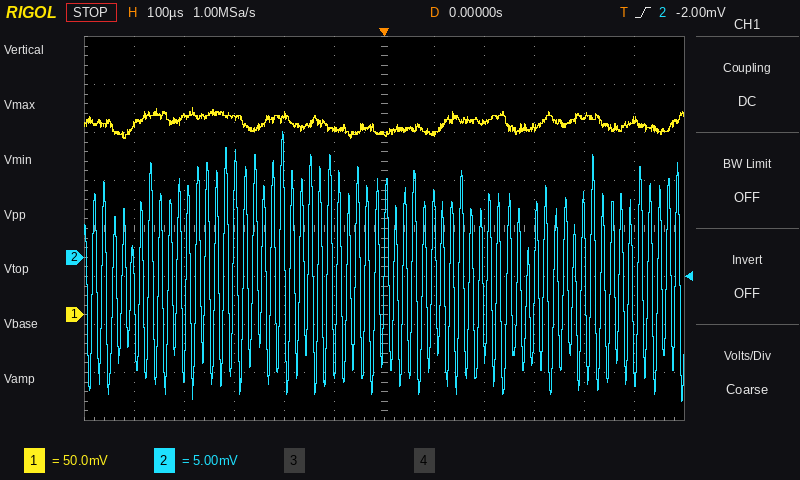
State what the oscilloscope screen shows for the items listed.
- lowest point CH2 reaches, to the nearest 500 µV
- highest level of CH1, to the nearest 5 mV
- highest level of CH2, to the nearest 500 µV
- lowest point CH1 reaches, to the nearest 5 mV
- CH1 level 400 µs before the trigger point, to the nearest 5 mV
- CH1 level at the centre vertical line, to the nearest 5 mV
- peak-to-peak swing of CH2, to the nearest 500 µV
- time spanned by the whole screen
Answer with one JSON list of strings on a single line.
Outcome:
["-15.0 mV", "215 mV", "13.0 mV", "185 mV", "205 mV", "190 mV", "28.0 mV", "1.2 ms"]
